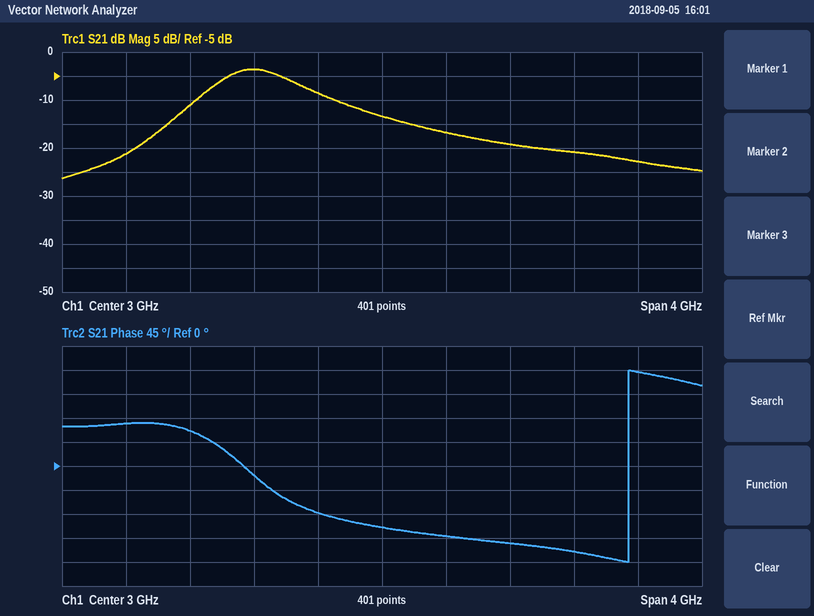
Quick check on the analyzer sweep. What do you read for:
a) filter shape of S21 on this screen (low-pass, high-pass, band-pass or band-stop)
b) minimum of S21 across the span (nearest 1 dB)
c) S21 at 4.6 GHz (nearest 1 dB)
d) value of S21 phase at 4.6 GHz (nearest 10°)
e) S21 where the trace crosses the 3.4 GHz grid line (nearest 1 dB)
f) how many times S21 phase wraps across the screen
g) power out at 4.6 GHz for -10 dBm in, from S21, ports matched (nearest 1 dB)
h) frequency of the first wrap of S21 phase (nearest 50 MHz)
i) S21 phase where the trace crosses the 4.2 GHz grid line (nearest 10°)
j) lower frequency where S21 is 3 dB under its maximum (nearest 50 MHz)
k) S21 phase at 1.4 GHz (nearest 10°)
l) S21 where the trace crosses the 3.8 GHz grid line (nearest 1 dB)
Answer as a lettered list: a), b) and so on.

a) band-pass
b) -26 dB
c) -23 dB
d) 180°
e) -17 dB
f) 1
g) -33 dBm
h) 4.55 GHz
i) -160°
j) 1.95 GHz
k) 80°
l) -19 dB
